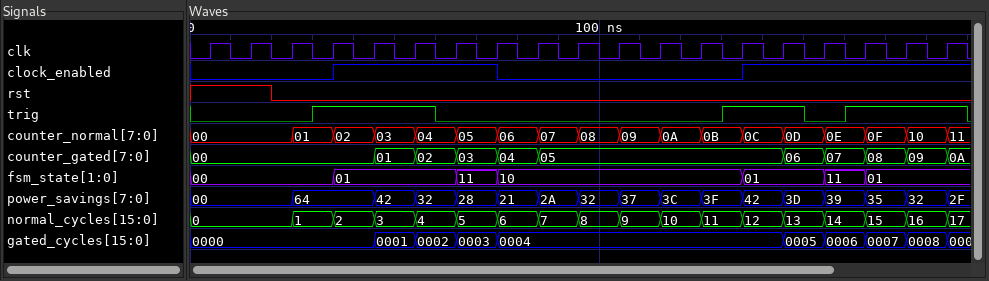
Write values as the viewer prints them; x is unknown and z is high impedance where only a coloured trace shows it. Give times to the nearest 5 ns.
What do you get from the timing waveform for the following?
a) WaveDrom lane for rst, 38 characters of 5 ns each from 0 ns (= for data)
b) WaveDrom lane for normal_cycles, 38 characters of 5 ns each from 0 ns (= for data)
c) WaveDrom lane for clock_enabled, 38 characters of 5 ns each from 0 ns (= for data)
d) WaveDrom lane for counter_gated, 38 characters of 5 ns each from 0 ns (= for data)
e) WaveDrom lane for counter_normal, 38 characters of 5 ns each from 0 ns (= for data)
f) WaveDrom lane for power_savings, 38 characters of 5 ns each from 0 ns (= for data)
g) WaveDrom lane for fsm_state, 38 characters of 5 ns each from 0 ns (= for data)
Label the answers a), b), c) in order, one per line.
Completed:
a) {name: 'rst', wave: '1...0.................................'}
b) {name: 'normal_cycles', wave: '=....=.=.=.=.=.=.=.=.=.=.=.=.=.=.=.=.=', data: '0 1 2 3 4 5 6 7 8 9 10 11 12 13 14 15 16 17'}
c) {name: 'clock_enabled', wave: '0......1.......0...........1..........'}
d) {name: 'counter_gated', wave: '=........=.=.=.=.=...........=.=.=.=.=', data: '00 01 02 03 04 05 06 07 08 09 0A'}
e) {name: 'counter_normal', wave: '=....=.=.=.=.=.=.=.=.=.=.=.=.=.=.=.=.=', data: '00 01 02 03 04 05 06 07 08 09 0A 0B 0C 0D 0E 0F 10 11'}
f) {name: 'power_savings', wave: '=....=...=.=.=.=.=.=.=.=.=.=.=.=.=.=.=', data: '00 64 42 32 28 21 2A 32 37 3C 3F 42 3D 39 35 32 2F'}
g) {name: 'fsm_state', wave: '=......=.....=.=...........=...=.=....', data: '00 01 11 10 01 11 01'}
